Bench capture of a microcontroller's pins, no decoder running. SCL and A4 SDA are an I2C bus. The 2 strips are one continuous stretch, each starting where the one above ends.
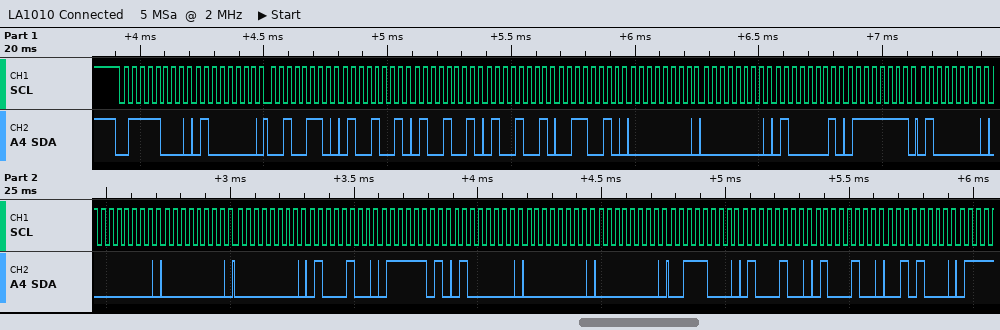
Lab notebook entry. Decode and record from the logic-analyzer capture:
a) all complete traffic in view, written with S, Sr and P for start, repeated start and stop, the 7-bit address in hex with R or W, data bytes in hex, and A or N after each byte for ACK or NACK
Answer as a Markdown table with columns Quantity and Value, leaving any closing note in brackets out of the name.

| Quantity | Value |
|---|---|
| all complete traffic in view, written with S, Sr and P for start, repeated start and stop, the 7-bit address in hex with R or W, data bytes in hex, and A or N after each byte for ACK or NACK | S 3CW A 40 A 26 A 49 A 49 A 49 A 32 A 00 A 00 A 41 A 7F A 40 A 00 A 00 A 00 A 44 A 7D A 40 A 00 A 00 A 38 A 44 A 44 A 28 A |
